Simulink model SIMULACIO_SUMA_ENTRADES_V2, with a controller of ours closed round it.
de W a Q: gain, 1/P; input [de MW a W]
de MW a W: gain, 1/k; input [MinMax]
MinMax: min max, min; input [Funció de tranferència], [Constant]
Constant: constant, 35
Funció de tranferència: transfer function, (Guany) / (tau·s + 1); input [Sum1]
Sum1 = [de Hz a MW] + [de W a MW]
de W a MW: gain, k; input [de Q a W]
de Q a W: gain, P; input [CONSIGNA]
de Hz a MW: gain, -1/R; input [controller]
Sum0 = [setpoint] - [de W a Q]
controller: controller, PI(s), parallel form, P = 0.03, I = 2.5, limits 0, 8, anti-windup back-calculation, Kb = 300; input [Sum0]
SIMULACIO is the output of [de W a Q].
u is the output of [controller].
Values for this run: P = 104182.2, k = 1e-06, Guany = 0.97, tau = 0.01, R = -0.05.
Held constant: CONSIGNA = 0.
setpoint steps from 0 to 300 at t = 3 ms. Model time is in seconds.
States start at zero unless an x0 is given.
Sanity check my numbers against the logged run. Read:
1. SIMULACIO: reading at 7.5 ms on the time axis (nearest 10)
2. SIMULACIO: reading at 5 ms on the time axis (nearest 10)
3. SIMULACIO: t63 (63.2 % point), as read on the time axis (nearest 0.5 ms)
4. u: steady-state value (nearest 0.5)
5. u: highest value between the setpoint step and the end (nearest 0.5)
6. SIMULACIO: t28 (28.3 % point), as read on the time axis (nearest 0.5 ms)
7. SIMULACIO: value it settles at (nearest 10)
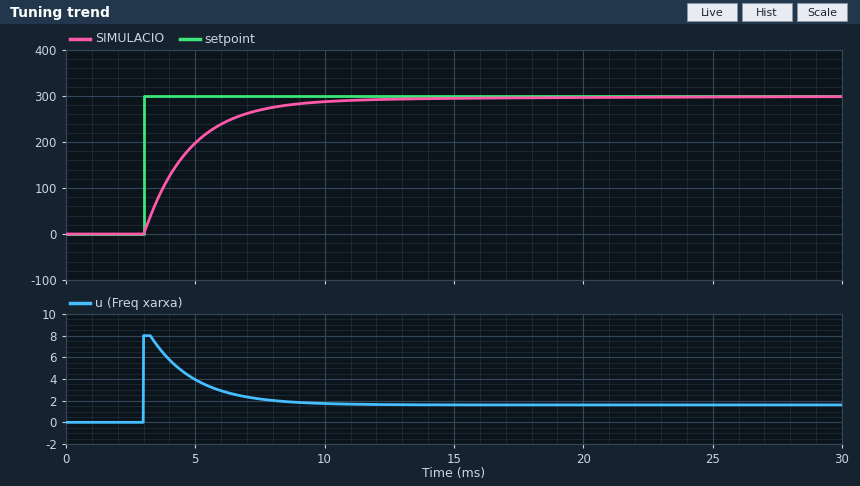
270
200
5.0 ms
1.5
8.0
3.5 ms
300
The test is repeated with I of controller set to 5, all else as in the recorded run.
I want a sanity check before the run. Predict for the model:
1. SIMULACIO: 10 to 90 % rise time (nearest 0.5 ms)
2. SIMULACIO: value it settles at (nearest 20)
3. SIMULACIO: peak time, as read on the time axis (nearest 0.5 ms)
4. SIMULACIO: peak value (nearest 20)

3.0 ms
300
11.0 ms
320
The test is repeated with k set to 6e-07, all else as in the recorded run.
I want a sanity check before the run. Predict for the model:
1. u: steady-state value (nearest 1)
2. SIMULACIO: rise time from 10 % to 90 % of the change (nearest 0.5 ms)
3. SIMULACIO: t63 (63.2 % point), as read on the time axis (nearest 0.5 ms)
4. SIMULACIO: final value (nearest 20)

1
2.5 ms
4.0 ms
300
